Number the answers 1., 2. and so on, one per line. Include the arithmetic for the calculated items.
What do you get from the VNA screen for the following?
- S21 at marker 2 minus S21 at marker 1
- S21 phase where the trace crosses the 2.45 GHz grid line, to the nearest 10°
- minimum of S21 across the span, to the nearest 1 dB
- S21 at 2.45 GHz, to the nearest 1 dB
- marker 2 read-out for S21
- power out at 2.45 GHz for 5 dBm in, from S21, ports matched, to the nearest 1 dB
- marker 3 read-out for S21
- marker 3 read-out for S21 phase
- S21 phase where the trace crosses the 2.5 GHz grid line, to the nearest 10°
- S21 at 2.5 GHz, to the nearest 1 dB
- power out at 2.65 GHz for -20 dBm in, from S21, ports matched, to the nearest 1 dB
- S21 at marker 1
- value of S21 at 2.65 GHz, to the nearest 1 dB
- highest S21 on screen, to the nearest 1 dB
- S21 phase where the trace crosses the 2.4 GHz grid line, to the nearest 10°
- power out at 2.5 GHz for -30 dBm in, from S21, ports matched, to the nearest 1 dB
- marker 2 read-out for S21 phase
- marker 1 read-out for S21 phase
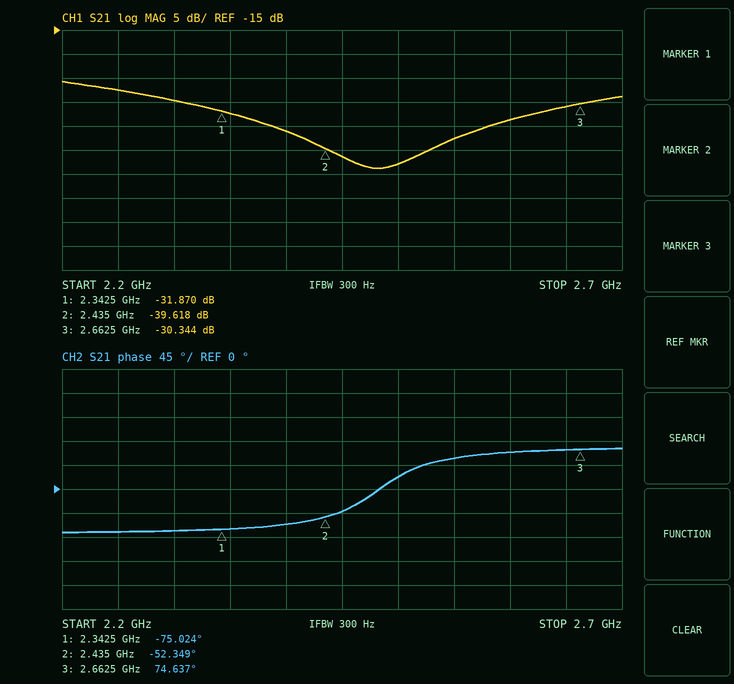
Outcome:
1. -39.618 − (-31.87) = -7.748 dB
2. -40°
3. -44 dB
4. -41 dB
5. -39.618 dB
6. 5 dBm + (-41 dB) = -36 dBm
7. -30.344 dB
8. 74.637°
9. 20°
10. -43 dB
11. -20 dBm + (-31 dB) = -51 dBm
12. -31.870 dB
13. -31 dB
14. -26 dB
15. -70°
16. -30 dBm + (-43 dB) = -73 dBm
17. -52.349°
18. -75.024°
